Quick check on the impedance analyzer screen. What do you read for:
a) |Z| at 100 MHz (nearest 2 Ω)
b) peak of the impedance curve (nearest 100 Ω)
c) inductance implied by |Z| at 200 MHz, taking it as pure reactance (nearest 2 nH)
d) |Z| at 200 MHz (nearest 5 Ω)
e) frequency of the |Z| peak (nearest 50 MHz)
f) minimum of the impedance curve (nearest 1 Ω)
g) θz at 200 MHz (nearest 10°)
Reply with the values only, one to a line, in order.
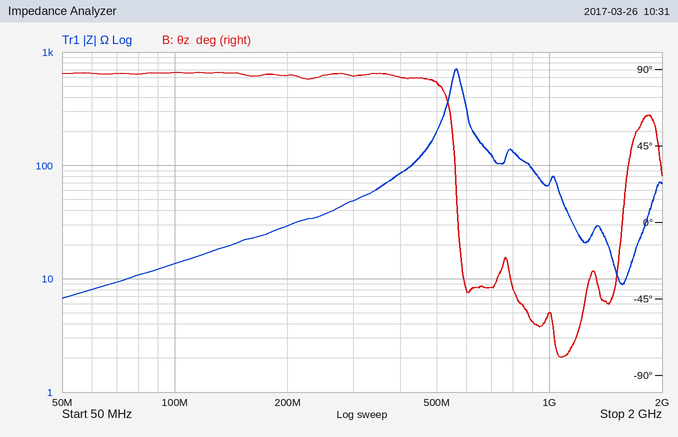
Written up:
14 Ω
700 Ω
24 nH
30 Ω
550 MHz
7 Ω
90°
